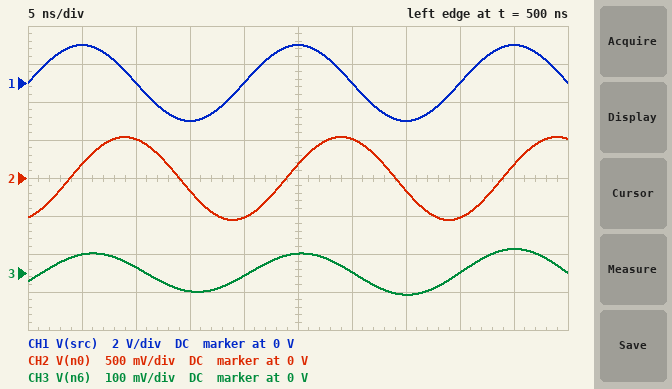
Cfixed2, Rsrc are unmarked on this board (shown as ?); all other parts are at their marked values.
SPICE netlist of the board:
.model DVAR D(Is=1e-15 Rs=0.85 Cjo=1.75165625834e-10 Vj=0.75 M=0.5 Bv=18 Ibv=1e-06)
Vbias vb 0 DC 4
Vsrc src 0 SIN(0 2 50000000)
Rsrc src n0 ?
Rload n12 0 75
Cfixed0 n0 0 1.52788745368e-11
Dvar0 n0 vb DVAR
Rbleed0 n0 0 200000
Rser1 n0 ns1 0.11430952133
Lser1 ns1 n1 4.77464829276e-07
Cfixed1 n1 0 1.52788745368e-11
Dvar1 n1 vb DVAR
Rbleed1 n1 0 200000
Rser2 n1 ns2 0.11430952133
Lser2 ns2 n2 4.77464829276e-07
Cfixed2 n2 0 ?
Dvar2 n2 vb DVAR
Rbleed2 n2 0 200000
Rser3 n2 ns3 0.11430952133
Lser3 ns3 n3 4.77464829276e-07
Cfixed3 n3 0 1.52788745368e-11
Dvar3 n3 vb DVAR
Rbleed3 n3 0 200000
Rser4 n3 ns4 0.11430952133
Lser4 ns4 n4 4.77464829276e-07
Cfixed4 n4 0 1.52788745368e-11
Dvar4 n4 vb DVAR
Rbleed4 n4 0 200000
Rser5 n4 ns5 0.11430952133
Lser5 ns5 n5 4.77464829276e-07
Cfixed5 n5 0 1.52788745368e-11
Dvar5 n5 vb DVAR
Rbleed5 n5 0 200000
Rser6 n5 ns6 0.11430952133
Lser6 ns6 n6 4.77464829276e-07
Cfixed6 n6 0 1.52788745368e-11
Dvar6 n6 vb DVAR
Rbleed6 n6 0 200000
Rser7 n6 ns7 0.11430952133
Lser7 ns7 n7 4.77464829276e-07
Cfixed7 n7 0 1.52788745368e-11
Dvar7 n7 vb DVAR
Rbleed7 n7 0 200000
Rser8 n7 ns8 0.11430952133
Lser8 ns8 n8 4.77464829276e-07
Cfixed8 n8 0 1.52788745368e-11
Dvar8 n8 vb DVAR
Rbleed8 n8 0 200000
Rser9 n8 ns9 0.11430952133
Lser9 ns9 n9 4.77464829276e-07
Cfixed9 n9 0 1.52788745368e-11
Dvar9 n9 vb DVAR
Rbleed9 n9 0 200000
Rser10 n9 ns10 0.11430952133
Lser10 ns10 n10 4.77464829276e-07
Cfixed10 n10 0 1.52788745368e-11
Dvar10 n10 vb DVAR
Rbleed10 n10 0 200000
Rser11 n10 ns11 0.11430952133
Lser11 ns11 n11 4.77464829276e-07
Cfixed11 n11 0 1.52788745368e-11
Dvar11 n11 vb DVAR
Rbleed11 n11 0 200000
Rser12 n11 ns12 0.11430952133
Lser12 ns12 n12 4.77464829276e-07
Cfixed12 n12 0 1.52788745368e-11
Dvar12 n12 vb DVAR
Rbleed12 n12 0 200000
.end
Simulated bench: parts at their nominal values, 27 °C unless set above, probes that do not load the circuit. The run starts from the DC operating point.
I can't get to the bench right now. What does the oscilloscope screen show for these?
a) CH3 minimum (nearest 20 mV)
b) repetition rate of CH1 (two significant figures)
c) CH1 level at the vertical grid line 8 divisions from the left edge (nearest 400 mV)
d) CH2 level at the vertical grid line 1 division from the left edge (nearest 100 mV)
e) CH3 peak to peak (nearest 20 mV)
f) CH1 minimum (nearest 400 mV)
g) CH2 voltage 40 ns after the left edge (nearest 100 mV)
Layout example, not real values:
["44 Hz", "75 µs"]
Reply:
["-60 mV", "50 MHz", "0 V", "200 mV", "120 mV", "-2.0 V", "-500 mV"]
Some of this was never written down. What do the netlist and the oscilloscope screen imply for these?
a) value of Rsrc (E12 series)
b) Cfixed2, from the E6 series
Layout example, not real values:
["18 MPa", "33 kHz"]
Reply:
["220 Ω", "47 pF"]
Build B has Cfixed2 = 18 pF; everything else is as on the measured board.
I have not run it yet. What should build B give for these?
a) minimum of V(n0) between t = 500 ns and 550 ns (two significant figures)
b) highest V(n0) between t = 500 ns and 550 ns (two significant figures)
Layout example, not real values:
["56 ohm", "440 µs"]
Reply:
["-570 mV", "560 mV"]
